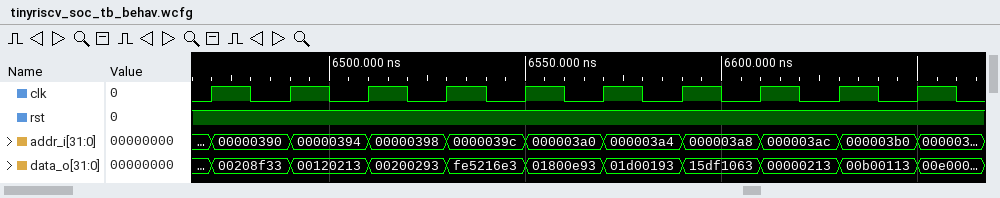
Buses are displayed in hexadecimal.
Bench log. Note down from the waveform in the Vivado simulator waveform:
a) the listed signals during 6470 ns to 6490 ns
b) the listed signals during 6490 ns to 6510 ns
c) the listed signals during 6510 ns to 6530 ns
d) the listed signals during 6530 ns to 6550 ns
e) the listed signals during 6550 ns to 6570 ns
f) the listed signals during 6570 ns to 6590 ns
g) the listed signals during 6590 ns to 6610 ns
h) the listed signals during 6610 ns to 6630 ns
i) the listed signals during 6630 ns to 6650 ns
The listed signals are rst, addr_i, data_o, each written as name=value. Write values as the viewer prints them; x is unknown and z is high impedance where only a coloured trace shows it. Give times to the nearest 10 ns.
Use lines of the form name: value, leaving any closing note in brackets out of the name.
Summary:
the listed signals during 6470 ns to 6490 ns: rst=1, addr_i=00000390, data_o=00208f33
the listed signals during 6490 ns to 6510 ns: rst=1, addr_i=00000394, data_o=00120213
the listed signals during 6510 ns to 6530 ns: rst=1, addr_i=00000398, data_o=00200293
the listed signals during 6530 ns to 6550 ns: rst=1, addr_i=0000039c, data_o=fe5216e3
the listed signals during 6550 ns to 6570 ns: rst=1, addr_i=000003a0, data_o=01800e93
the listed signals during 6570 ns to 6590 ns: rst=1, addr_i=000003a4, data_o=01d00193
the listed signals during 6590 ns to 6610 ns: rst=1, addr_i=000003a8, data_o=15df1063
the listed signals during 6610 ns to 6630 ns: rst=1, addr_i=000003ac, data_o=00000213
the listed signals during 6630 ns to 6650 ns: rst=1, addr_i=000003b0, data_o=00b00113
